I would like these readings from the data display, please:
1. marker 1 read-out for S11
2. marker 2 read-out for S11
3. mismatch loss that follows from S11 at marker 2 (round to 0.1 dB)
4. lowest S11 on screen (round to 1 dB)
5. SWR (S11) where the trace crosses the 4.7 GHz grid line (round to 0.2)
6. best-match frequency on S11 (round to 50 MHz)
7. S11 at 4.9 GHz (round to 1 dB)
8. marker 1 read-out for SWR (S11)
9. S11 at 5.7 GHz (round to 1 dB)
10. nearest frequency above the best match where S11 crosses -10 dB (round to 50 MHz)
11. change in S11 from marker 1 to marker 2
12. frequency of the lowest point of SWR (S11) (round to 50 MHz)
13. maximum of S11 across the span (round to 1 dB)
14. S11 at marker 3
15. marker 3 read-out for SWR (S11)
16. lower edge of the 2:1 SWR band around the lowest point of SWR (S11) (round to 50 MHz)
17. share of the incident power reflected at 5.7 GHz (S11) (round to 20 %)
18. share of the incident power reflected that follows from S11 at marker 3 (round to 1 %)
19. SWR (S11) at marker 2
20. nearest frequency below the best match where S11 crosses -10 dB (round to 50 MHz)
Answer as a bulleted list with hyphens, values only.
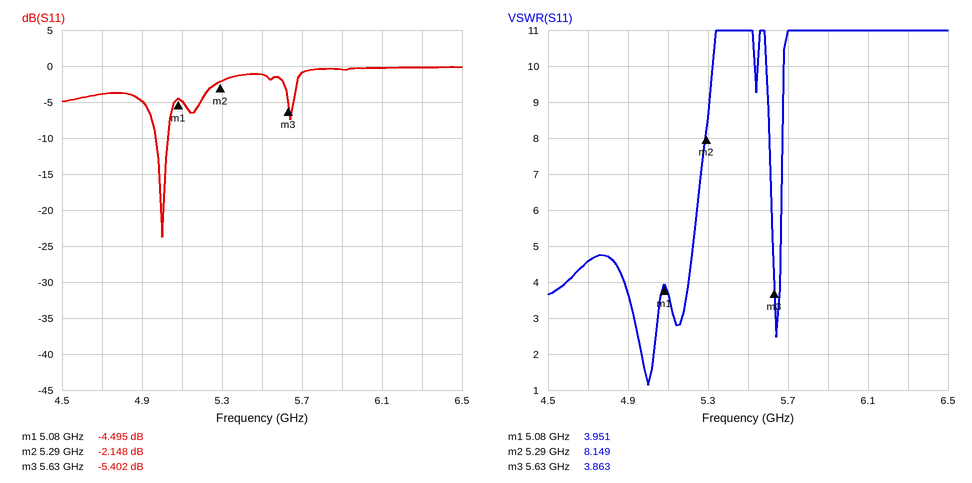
- -4.495 dB
- -2.148 dB
- 4.1 dB
- -24 dB
- 4.6
- 5.00 GHz
- -5 dB
- 3.951
- -1 dB
- 5.05 GHz
- 2.347 dB
- 5.00 GHz
- 0 dB
- -5.402 dB
- 3.863
- 4.95 GHz
- 80 %
- 29 %
- 8.149
- 4.95 GHz
